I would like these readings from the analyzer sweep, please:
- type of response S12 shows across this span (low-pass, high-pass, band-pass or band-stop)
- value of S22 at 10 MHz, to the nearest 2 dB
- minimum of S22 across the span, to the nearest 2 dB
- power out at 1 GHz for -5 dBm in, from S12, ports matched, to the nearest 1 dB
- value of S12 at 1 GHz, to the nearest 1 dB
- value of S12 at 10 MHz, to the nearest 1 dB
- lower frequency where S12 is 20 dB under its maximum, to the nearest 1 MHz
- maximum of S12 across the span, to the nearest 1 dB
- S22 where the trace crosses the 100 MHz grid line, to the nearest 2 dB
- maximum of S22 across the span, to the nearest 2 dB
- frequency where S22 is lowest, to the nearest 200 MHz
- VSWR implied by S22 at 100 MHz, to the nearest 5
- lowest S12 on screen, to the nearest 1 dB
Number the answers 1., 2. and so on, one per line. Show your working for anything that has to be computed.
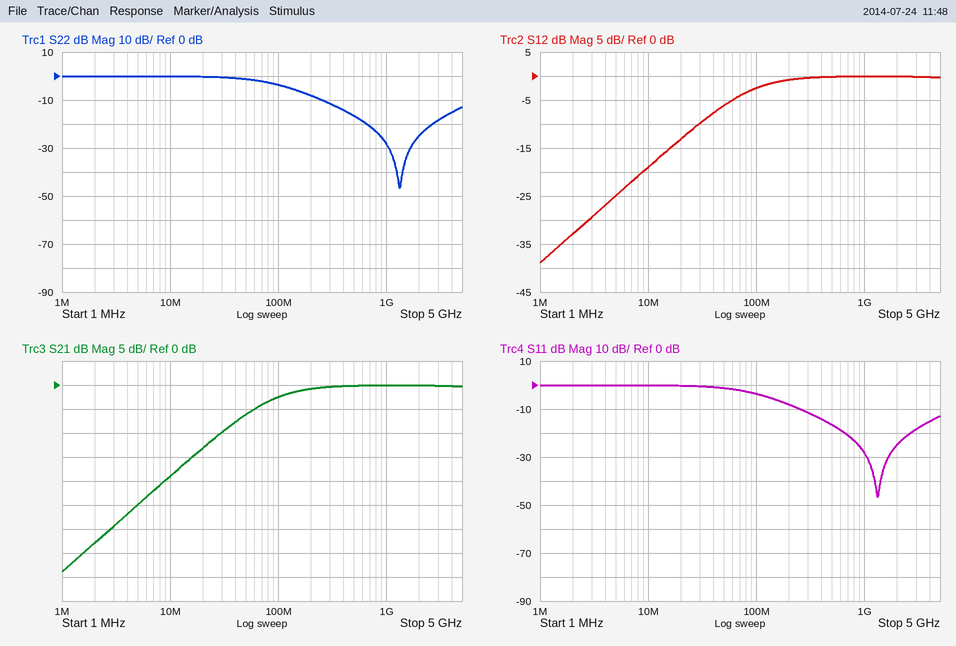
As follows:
1. high-pass
2. 0 dB
3. -46 dB
4. -5 dBm + (0 dB) = -5 dBm
5. 0 dB
6. -19 dB
7. 9 MHz
8. 0 dB
9. -4 dB
10. 0 dB
11. 1.4 GHz
12. |Γ| = 10^(-4/20) = 0.6310; VSWR = (1 + 0.6310)/(1 − 0.6310) ≈ 4.42, so 5 to the nearest 5
13. -39 dB
